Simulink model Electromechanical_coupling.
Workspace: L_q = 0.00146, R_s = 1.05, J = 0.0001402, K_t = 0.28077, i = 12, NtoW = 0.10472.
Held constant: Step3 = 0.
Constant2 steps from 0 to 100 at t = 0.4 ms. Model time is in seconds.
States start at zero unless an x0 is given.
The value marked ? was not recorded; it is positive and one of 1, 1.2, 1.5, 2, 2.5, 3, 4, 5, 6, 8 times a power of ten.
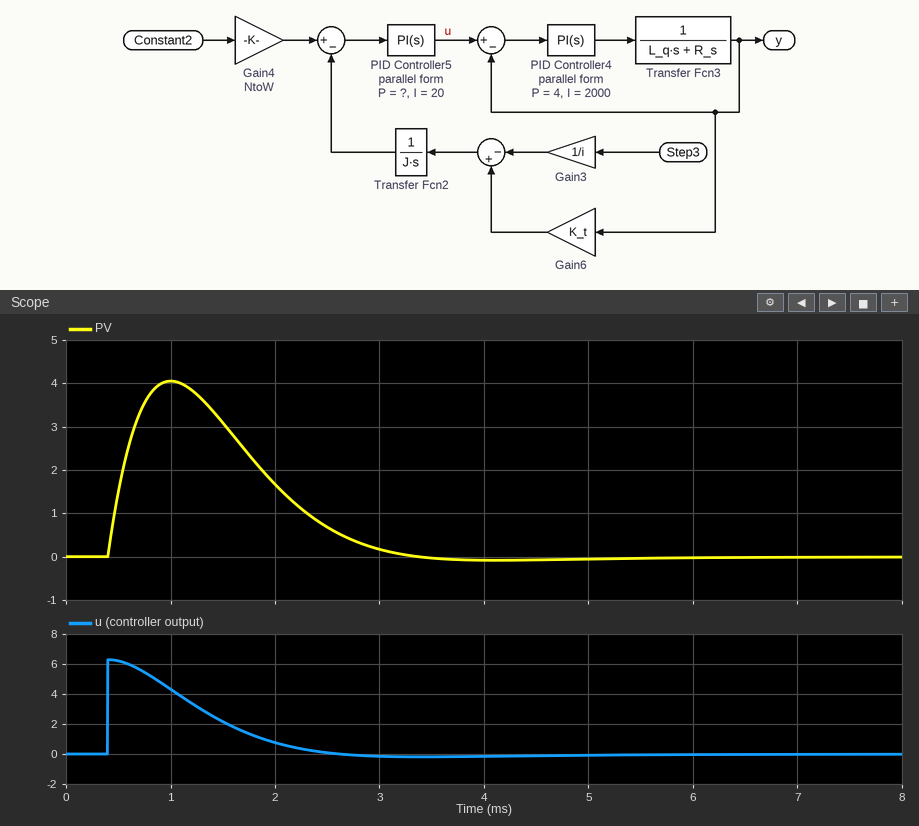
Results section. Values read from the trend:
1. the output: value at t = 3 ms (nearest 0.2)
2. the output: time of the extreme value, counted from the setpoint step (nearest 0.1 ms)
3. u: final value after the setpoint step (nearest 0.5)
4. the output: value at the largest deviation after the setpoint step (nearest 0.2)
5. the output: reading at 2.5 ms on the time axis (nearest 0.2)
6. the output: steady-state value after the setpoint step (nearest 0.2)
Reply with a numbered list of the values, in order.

1. 0.2
2. 0.6 ms
3. 0.0
4. 4.0
5. 0.6
6. 0.0
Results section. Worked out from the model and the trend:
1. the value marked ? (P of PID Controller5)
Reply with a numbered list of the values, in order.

1. 0.6
